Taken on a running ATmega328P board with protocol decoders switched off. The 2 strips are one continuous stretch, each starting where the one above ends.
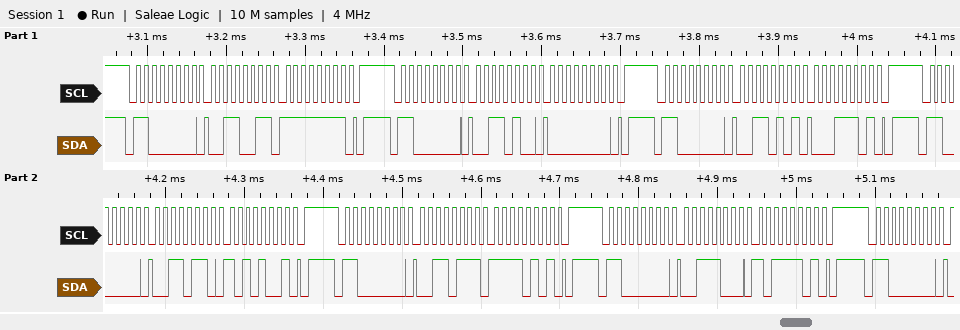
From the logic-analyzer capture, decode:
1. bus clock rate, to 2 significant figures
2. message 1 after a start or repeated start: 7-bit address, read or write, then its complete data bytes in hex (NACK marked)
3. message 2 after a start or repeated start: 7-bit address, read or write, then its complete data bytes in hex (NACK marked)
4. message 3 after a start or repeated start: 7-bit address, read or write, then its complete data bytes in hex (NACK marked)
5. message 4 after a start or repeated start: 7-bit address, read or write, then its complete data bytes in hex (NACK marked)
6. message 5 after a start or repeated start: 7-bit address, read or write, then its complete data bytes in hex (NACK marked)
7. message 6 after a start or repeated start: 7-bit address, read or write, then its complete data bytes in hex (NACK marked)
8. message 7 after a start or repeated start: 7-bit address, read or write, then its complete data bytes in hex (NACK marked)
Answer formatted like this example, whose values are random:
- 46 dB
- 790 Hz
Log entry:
- 100 kHz
- 0x60 write: 33 FF
- 0x60 write: 34 00
- 0x60 write: 35 1D
- 0x60 write: 36 A9
- 0x60 write: 37 F5
- 0x60 write: 38 BD
- 0x60 write
